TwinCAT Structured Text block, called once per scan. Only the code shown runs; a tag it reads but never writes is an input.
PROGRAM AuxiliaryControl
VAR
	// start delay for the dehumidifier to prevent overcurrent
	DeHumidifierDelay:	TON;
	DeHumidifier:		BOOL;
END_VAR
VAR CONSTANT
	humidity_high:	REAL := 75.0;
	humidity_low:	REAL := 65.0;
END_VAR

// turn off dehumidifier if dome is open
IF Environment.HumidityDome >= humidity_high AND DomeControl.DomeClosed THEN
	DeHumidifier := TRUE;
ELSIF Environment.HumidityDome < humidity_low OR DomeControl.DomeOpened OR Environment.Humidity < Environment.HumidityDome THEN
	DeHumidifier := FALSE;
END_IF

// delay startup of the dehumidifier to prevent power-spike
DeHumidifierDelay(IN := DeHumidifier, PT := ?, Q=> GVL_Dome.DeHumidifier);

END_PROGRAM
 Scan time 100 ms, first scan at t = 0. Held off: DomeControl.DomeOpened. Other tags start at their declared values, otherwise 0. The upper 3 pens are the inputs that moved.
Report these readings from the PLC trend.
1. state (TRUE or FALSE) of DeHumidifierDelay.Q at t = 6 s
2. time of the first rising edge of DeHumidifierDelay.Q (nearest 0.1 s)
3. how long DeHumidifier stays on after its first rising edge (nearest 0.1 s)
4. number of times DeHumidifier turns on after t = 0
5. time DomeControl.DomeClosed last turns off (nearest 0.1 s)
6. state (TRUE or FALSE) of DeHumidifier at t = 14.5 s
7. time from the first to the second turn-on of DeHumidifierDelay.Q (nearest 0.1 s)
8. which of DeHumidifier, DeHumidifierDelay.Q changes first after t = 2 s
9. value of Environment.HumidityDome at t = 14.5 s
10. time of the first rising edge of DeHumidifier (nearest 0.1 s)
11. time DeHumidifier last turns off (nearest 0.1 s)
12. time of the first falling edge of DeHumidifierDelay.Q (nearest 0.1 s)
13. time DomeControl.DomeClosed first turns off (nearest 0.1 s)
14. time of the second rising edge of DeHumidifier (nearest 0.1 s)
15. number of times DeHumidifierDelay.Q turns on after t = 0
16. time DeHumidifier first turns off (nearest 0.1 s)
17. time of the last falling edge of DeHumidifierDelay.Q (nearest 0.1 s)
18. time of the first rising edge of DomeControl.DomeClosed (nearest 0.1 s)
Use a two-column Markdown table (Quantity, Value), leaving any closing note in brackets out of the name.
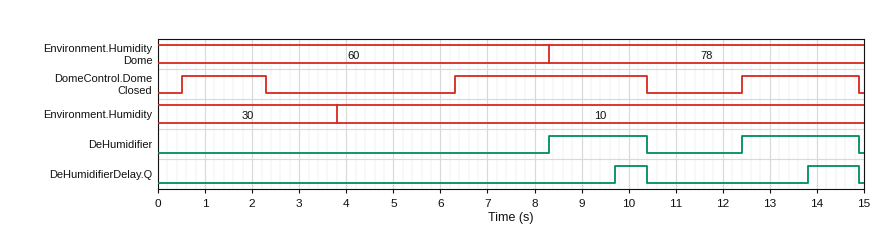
| Quantity | Value |
|---|---|
| state (TRUE or FALSE) of DeHumidifierDelay.Q at t = 6 s | FALSE |
| time of the first rising edge of DeHumidifierDelay.Q | 9.7 s |
| how long DeHumidifier stays on after its first rising edge | 2.1 s |
| number of times DeHumidifier turns on after t = 0 | 2 |
| time DomeControl.DomeClosed last turns off | 14.9 s |
| state (TRUE or FALSE) of DeHumidifier at t = 14.5 s | TRUE |
| time from the first to the second turn-on of DeHumidifierDelay.Q | 4.1 s |
| which of DeHumidifier, DeHumidifierDelay.Q changes first after t = 2 s | DeHumidifier |
| value of Environment.HumidityDome at t = 14.5 s | 78 |
| time of the first rising edge of DeHumidifier | 8.3 s |
| time DeHumidifier last turns off | 14.9 s |
| time of the first falling edge of DeHumidifierDelay.Q | 10.4 s |
| time DomeControl.DomeClosed first turns off | 2.3 s |
| time of the second rising edge of DeHumidifier | 12.4 s |
| number of times DeHumidifierDelay.Q turns on after t = 0 | 2 |
| time DeHumidifier first turns off | 10.4 s |
| time of the last falling edge of DeHumidifierDelay.Q | 14.9 s |
| time of the first rising edge of DomeControl.DomeClosed | 0.5 s |
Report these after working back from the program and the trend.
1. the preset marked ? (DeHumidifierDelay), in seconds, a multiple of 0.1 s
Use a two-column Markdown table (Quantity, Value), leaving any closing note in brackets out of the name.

| Quantity | Value |
|---|---|
| the preset marked ? (DeHumidifierDelay), in seconds, a multiple of 0.1 s | 1.4 s |
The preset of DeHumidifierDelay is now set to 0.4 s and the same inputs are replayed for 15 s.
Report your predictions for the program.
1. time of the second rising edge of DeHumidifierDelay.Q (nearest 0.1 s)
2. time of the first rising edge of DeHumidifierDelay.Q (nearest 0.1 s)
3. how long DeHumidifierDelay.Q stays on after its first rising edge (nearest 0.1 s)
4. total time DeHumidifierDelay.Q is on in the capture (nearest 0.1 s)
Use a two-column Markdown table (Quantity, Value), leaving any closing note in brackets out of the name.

| Quantity | Value |
|---|---|
| time of the second rising edge of DeHumidifierDelay.Q | 12.8 s |
| time of the first rising edge of DeHumidifierDelay.Q | 8.7 s |
| how long DeHumidifierDelay.Q stays on after its first rising edge | 1.7 s |
| total time DeHumidifierDelay.Q is on in the capture | 3.8 s |
